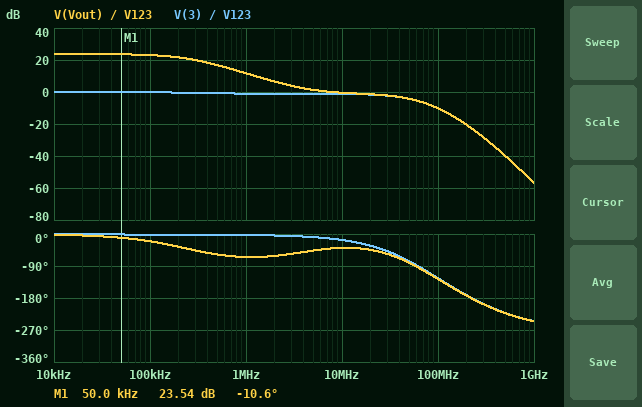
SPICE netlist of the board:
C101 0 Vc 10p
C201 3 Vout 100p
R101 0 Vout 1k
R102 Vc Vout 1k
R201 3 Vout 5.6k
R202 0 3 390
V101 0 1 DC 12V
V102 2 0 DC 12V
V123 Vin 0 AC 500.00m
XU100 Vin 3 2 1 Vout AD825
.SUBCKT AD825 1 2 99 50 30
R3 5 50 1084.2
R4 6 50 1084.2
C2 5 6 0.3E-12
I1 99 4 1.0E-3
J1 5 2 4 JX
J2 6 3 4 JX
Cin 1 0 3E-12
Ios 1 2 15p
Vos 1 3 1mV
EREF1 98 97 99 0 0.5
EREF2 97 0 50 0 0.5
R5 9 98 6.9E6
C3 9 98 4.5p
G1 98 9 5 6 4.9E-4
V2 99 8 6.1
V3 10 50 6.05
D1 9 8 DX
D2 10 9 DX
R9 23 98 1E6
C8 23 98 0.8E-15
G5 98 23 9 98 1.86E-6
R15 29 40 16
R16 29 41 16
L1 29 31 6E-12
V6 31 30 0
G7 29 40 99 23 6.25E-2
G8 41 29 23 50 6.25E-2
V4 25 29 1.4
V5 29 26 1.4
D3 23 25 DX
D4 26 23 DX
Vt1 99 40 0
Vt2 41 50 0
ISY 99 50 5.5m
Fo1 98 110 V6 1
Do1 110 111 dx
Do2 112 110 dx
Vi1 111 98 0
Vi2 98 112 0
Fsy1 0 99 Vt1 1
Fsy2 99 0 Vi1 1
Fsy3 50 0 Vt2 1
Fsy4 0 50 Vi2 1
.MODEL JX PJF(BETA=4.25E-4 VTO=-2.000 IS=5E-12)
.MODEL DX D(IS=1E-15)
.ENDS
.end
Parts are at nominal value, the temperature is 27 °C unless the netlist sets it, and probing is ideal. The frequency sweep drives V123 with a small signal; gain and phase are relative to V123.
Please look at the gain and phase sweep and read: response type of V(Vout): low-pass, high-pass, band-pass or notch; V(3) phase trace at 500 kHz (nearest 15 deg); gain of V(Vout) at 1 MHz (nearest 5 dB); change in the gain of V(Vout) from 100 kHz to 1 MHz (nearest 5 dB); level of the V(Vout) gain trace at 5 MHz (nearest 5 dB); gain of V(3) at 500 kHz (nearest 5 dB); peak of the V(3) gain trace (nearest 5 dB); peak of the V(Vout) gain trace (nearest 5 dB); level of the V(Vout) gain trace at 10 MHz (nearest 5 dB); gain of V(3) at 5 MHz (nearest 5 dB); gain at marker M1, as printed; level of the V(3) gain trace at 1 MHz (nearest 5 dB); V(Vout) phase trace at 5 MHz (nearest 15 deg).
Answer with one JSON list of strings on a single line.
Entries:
["low-pass", "0 deg", "10 dB", "-10 dB", "0 dB", "0 dB", "0 dB", "25 dB", "0 dB", "0 dB", "23.54 dB", "0 dB", "-45 deg"]
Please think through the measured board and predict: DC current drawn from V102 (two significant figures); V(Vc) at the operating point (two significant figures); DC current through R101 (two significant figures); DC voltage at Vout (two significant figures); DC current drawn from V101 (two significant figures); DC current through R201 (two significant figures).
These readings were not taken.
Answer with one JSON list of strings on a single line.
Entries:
["6.5 mA", "-15 mV", "15 µA", "-15 mV", "6.5 mA", "2.6 µA"]
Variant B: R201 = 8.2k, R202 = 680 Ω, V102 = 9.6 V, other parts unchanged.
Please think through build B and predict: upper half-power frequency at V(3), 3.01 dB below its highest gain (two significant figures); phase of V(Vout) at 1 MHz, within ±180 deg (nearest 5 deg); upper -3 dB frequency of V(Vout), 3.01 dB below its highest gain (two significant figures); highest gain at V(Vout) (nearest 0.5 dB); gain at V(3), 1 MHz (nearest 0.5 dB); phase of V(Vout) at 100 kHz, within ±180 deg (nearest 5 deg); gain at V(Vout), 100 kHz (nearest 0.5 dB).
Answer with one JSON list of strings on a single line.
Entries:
["41 MHz", "-60 deg", "180 kHz", "22.5 dB", "-0.5 dB", "-25 deg", "21.0 dB"]
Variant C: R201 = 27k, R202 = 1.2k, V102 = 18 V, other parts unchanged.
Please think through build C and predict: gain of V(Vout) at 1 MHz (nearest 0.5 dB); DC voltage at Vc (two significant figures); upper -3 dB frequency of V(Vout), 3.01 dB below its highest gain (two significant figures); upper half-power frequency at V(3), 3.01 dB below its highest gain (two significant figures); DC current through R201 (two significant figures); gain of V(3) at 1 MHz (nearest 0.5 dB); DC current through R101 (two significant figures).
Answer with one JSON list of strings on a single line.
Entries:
["4.5 dB", "-12 mV", "57 kHz", "43 MHz", "430 nA", "-0.5 dB", "12 µA"]
